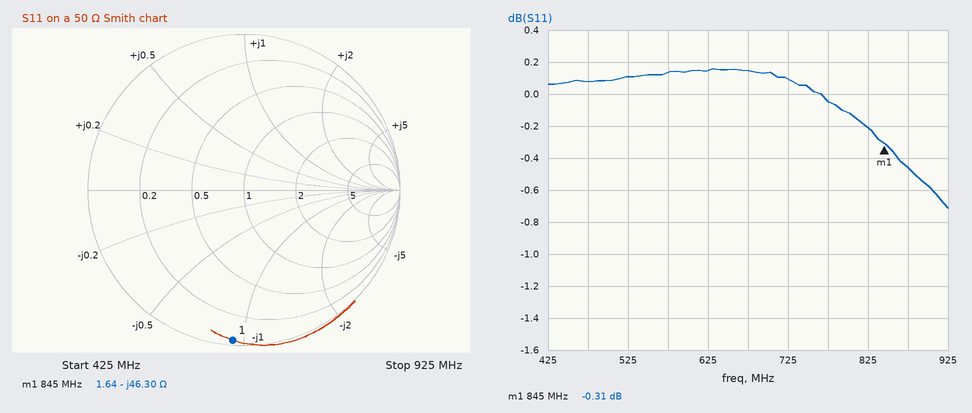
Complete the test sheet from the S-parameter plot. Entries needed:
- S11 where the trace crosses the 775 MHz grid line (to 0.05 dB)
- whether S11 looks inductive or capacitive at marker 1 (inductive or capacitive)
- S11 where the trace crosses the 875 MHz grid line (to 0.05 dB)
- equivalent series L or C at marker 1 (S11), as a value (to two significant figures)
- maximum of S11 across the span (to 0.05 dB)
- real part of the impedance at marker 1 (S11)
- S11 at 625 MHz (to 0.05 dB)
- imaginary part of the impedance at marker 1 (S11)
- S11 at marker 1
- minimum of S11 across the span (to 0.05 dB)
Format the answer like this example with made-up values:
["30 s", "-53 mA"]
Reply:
["-0.05 dB", "capacitive", "-0.45 dB", "4.1 pF", "0.15 dB", "1.64 Ω", "0.15 dB", "-46.30 Ω", "-0.31 dB", "-0.70 dB"]
